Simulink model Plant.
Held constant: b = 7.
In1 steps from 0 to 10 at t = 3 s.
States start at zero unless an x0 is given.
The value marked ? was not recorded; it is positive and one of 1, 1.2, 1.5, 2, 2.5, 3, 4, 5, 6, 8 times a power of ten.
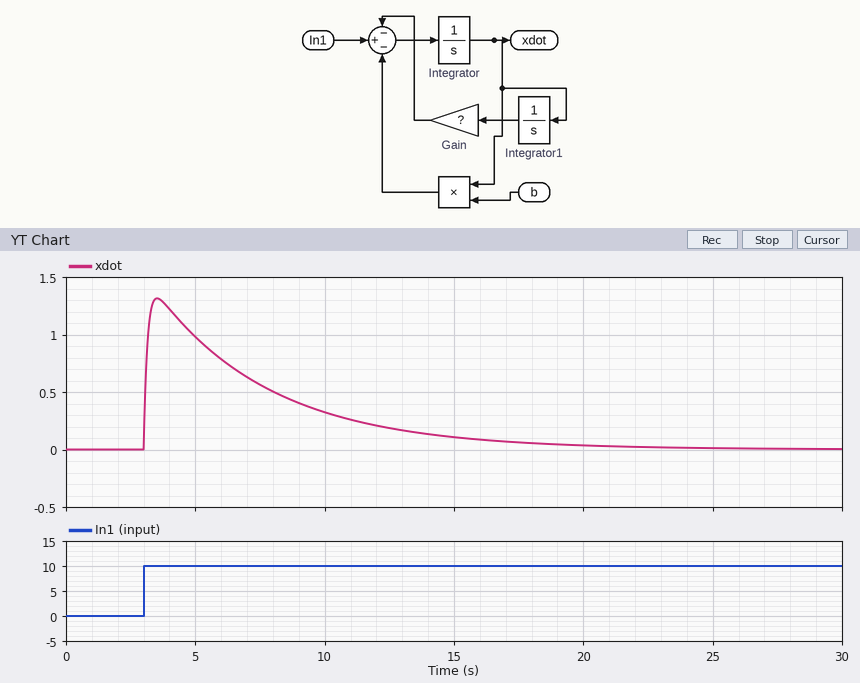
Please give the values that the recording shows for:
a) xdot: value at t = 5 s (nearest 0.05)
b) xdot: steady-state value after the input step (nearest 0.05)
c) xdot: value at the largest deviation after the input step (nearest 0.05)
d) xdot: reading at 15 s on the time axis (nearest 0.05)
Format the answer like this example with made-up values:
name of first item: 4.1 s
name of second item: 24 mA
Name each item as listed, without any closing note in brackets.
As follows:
xdot: value at t = 5 s: 1.00
xdot: steady-state value after the input step: 0.00
xdot: value at the largest deviation after the input step: 1.30
xdot: reading at 15 s on the time axis: 0.10
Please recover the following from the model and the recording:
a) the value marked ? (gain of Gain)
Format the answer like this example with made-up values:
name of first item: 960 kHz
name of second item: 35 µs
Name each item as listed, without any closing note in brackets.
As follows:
the value marked ?: 1.5
